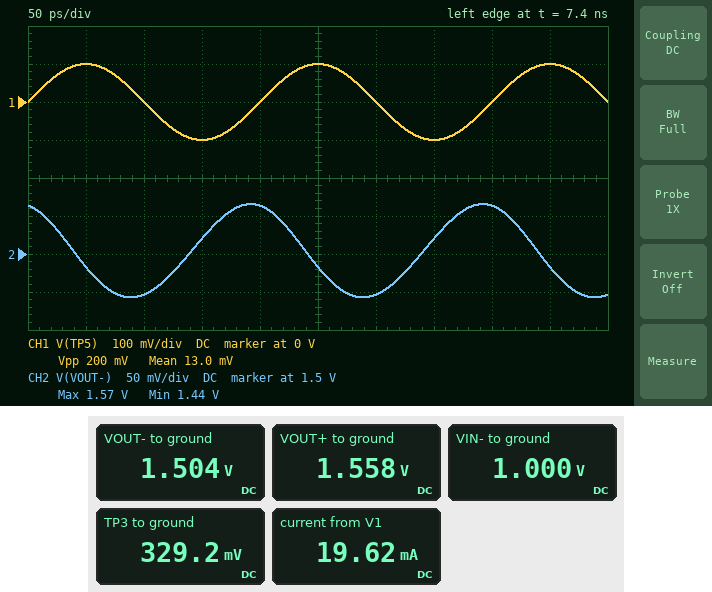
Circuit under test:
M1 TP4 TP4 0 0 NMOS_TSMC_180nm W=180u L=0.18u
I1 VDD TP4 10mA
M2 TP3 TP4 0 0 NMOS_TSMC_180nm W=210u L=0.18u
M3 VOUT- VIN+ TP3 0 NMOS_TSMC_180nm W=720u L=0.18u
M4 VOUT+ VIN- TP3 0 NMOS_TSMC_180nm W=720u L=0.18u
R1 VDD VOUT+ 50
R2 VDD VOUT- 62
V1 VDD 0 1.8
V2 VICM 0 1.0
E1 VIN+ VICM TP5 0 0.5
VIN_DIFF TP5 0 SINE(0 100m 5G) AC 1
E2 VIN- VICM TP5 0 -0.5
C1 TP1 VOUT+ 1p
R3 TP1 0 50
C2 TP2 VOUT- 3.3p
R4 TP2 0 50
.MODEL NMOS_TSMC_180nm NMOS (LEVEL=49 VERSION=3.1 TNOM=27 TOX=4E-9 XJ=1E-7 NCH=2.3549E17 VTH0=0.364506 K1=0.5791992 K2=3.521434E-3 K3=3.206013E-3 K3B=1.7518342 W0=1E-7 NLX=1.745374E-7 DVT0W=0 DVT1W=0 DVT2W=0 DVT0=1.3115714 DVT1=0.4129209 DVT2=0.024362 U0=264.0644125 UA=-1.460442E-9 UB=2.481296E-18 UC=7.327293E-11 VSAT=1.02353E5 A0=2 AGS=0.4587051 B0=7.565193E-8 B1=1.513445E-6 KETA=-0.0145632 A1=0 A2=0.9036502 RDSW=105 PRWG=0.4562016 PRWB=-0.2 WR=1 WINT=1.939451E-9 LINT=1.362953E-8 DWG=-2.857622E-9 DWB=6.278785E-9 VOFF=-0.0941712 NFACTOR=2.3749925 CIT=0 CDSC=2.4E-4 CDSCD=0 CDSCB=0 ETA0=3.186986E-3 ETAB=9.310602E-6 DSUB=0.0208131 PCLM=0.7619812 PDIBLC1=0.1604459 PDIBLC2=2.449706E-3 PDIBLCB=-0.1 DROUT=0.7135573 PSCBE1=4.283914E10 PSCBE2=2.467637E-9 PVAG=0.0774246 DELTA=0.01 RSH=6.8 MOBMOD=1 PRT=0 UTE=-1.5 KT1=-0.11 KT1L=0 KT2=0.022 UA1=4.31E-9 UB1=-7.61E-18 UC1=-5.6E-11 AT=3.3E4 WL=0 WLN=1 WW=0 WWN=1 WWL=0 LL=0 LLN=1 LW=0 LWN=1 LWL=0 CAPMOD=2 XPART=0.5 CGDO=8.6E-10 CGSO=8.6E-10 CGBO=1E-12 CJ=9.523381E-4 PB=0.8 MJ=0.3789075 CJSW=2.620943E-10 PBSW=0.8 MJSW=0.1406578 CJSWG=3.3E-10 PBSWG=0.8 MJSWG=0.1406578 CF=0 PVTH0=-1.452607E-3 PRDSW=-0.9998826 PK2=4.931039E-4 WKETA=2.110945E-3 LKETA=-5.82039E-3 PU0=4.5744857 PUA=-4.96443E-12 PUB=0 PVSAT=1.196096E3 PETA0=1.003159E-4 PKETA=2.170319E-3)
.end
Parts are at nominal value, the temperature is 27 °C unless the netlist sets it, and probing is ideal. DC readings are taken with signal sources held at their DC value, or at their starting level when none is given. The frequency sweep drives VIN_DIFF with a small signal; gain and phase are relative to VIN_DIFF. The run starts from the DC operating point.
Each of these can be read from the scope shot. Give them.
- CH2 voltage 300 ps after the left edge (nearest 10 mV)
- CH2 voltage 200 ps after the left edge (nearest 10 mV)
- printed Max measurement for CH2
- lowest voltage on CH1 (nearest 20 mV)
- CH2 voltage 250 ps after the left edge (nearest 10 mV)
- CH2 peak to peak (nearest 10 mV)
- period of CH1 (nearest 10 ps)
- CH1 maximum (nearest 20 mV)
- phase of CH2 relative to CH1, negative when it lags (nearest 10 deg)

1.45 V
1.56 V
1.57 V
-100 mV
1.48 V
120 mV
200 ps
100 mV
110 deg
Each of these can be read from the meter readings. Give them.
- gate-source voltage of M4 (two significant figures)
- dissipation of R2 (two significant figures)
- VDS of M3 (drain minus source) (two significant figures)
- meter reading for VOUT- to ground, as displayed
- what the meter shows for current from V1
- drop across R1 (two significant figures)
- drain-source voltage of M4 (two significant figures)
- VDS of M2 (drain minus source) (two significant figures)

670 mV
1.4 mW
1.2 V
1.504 V
19.62 mA
240 mV
1.2 V
330 mV
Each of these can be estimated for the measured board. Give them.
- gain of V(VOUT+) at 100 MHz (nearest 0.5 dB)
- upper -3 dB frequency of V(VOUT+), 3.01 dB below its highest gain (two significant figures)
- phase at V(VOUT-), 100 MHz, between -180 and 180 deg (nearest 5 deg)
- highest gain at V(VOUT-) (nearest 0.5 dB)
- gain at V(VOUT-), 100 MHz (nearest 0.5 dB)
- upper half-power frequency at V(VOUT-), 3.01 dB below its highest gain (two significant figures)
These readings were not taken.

1.0 dB
1.6 GHz
170 deg
3.0 dB
3.0 dB
530 MHz
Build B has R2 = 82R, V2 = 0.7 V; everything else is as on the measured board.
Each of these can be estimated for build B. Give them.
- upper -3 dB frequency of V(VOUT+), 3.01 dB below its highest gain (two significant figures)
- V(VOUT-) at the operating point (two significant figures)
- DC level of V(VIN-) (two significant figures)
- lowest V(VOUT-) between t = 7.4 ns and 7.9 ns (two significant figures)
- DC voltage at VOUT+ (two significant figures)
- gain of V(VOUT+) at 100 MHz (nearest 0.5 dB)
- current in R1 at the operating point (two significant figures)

1.7 GHz
1.6 V
700 mV
1.5 V
1.7 V
-1.5 dB
2.7 mA
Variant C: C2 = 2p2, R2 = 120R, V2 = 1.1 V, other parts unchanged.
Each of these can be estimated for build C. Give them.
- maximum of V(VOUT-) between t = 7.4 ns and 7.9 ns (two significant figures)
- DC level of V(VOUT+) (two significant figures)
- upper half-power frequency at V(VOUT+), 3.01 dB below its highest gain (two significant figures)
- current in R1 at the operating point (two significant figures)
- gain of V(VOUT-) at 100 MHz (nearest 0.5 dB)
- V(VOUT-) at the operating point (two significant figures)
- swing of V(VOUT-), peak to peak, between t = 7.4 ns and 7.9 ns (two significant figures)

1.3 V
1.5 V
1.8 GHz
5.2 mA
8.5 dB
1.2 V
140 mV
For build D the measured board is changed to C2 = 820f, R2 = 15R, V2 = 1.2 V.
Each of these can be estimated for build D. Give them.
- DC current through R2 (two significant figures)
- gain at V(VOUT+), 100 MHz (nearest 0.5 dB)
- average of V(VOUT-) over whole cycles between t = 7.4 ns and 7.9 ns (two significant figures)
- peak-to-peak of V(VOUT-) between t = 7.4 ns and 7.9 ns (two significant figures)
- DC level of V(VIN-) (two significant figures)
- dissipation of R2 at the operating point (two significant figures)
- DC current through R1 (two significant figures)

5.3 mA
1.5 dB
1.7 V
65 mV
1.2 V
420 µW
5.1 mA
